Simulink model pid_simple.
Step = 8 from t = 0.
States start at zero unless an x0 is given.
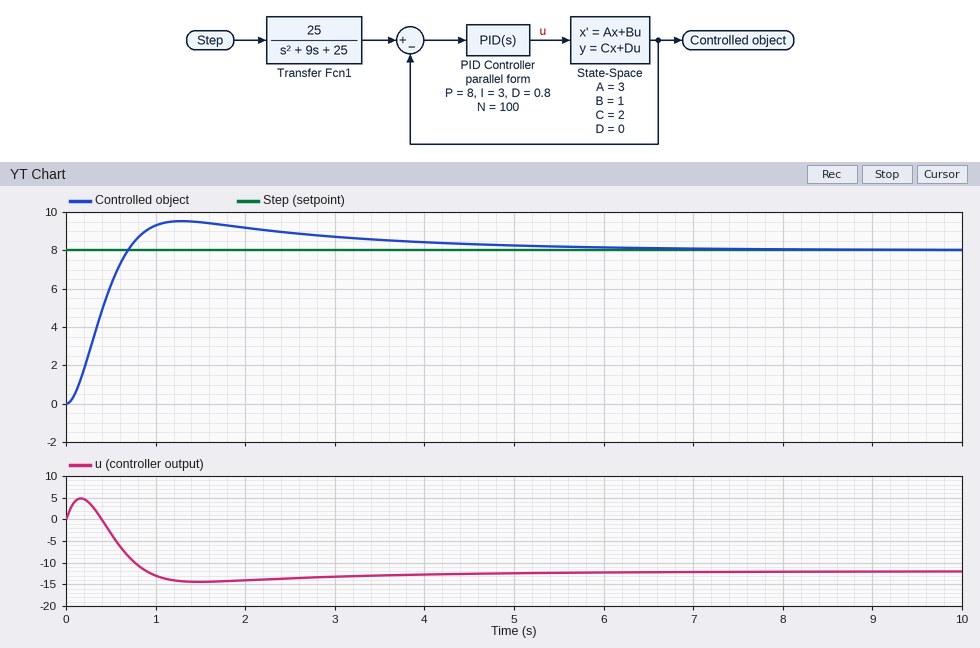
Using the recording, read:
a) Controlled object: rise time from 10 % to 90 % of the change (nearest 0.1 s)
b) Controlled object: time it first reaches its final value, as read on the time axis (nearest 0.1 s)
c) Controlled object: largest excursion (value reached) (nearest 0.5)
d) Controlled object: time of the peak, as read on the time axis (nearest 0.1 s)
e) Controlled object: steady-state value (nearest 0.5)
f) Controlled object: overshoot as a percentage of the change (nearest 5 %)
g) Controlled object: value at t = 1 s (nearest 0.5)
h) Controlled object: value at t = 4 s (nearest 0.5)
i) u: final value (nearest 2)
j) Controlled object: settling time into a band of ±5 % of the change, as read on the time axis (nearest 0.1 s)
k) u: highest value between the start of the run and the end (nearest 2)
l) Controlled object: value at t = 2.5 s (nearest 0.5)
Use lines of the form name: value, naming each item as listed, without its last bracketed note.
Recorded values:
Controlled object: rise time from 10 % to 90 % of the change: 0.5 s
Controlled object: time it first reaches its final value, as read on the time axis: 0.7 s
Controlled object: largest excursion (value reached): 9.5
Controlled object: time of the peak, as read on the time axis: 1.3 s
Controlled object: steady-state value: 8.0
Controlled object: overshoot as a percentage of the change: 20 %
Controlled object: value at t = 1 s: 9.5
Controlled object: value at t = 4 s: 8.5
u: final value: -12
Controlled object: settling time into a band of ±5 % of the change, as read on the time axis: 4.1 s
u: highest value between the start of the run and the end: 4
Controlled object: value at t = 2.5 s: 9.0
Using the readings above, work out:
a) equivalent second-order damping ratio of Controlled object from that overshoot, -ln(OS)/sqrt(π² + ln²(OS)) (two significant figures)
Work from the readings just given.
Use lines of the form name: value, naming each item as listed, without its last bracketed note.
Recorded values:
equivalent second-order damping ratio of Controlled object from that overshoot, -ln(OS)/sqrt(π² + ln²(OS)): 0.46
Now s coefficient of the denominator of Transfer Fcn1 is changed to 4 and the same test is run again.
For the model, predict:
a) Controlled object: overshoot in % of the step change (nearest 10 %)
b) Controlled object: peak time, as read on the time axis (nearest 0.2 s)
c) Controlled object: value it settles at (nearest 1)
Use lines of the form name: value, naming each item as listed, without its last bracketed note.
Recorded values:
Controlled object: overshoot in % of the step change: 40 %
Controlled object: peak time, as read on the time axis: 0.8 s
Controlled object: value it settles at: 8
